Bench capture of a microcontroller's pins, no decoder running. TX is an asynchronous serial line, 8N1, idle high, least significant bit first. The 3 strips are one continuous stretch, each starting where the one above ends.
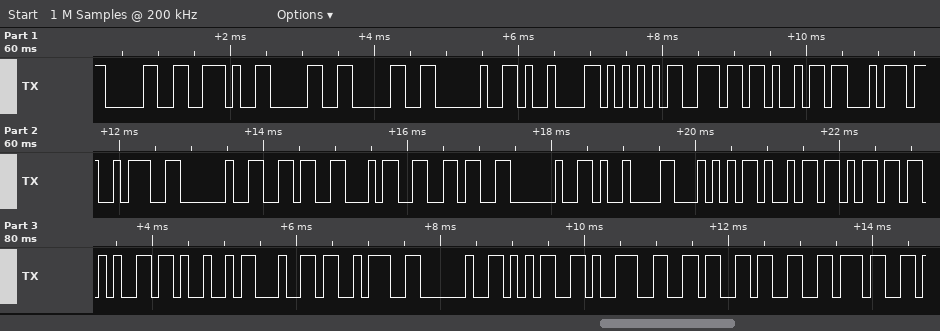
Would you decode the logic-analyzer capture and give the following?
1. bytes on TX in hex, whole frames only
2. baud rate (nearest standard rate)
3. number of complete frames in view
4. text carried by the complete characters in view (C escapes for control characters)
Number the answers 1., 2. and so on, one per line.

1. 30 2E 30 30 20 09 55 6E 69 74 3A 20 36 34 36 20 09 54 69 6D 65 49 64 3A 20 35 39 36 33 37
2. 9600 baud
3. 30
4. "0.00 \tUnit: 646 \tTimeId: 59637"
